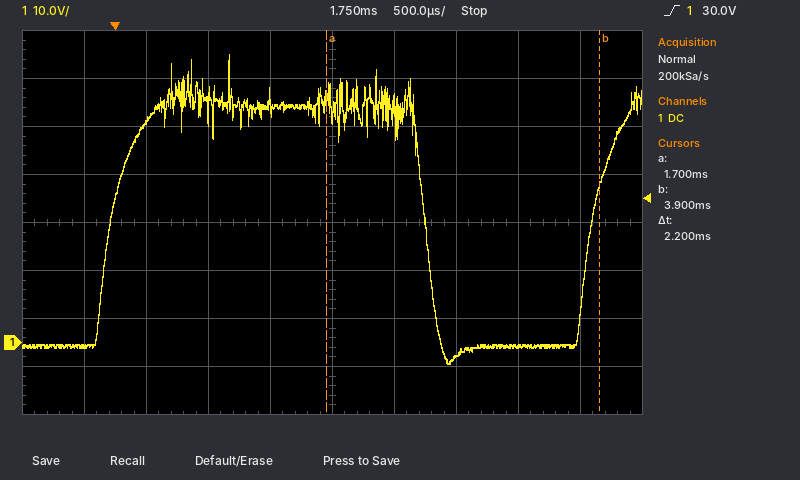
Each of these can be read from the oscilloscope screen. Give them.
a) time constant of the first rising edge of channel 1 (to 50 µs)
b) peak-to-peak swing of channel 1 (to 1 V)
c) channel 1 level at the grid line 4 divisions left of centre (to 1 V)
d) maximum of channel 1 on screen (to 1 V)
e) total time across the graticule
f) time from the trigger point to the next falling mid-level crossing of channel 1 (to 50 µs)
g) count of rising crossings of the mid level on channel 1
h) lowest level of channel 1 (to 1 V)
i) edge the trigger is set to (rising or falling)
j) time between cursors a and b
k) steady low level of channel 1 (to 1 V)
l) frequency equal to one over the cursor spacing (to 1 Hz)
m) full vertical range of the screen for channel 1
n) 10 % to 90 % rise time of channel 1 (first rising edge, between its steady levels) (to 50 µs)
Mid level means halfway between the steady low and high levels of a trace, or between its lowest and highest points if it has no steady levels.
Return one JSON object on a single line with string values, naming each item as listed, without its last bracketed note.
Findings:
{"time constant of the first rising edge of channel 1": "150 µs", "peak-to-peak swing of channel 1": "64 V", "channel 1 level at the grid line 4 divisions left of centre": "-1 V", "maximum of channel 1 on screen": "60 V", "total time across the graticule": "5 ms", "time from the trigger point to the next falling mid-level crossing of channel 1": "2.50 ms", "count of rising crossings of the mid level on channel 1": "2", "lowest level of channel 1": "-4 V", "edge the trigger is set to": "rising", "time between cursors a and b": "2.2 ms", "steady low level of channel 1": "-1 V", "frequency equal to one over the cursor spacing": "455 Hz", "full vertical range of the screen for channel 1": "80 V", "10 % to 90 % rise time of channel 1 (first rising edge, between its steady levels)": "350 µs"}
